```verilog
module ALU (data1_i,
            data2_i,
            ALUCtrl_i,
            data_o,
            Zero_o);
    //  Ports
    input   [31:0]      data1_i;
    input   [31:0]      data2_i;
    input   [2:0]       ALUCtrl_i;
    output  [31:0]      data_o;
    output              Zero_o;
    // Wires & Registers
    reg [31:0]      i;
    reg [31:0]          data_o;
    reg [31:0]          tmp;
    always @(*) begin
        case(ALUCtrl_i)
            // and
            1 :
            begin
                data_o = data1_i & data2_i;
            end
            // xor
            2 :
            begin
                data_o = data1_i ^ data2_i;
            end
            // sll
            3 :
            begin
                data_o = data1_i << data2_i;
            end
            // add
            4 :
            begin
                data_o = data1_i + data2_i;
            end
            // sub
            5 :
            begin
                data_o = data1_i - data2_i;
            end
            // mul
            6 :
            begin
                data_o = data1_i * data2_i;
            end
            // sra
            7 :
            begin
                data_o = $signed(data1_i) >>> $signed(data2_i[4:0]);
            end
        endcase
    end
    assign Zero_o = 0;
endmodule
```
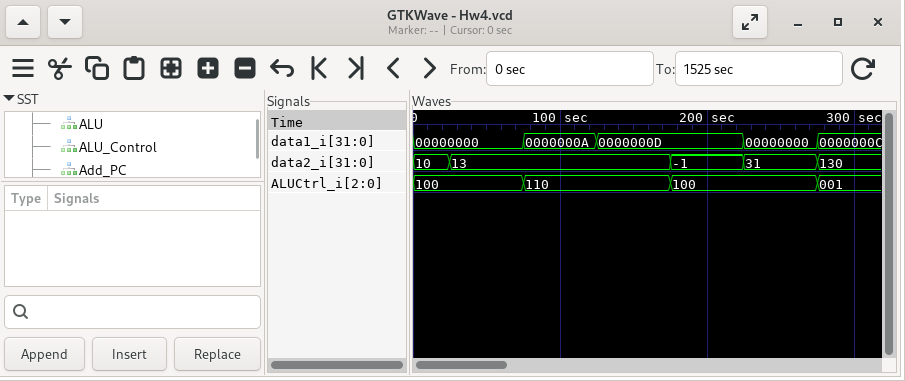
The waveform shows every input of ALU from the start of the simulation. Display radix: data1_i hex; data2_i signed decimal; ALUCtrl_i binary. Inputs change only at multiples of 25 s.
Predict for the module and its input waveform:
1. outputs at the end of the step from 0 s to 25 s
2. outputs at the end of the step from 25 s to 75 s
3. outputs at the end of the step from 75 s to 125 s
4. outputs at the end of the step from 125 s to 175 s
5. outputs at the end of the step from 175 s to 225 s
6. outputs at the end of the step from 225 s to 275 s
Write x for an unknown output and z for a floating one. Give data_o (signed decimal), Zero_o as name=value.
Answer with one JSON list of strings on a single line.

["data_o=10, Zero_o=0", "data_o=13, Zero_o=0", "data_o=130, Zero_o=0", "data_o=169, Zero_o=0", "data_o=12, Zero_o=0", "data_o=31, Zero_o=0"]
